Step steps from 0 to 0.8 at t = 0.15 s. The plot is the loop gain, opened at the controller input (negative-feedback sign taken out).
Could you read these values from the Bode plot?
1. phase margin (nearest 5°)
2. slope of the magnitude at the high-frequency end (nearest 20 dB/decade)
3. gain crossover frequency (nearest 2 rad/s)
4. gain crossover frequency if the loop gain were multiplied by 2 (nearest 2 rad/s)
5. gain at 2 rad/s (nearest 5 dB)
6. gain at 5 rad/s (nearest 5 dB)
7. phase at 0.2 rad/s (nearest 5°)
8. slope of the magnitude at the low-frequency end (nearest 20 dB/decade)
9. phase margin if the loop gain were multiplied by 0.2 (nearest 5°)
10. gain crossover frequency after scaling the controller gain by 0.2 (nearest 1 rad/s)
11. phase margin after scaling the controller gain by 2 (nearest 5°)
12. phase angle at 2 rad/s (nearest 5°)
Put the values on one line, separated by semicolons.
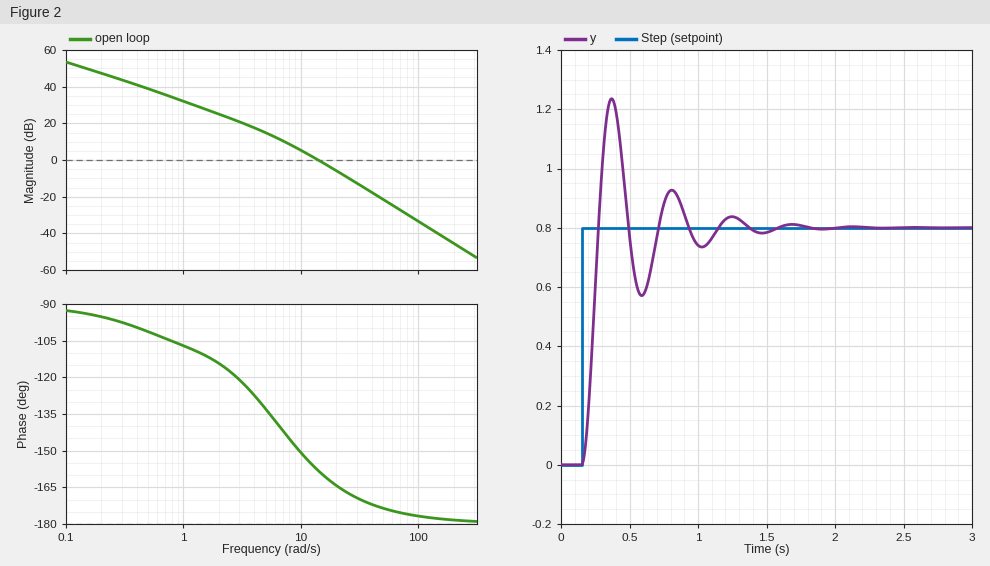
20°; -40 dB/decade; 14 rad/s; 20 rad/s; 25 dB; 15 dB; -95°; -20 dB/decade; 45°; 5 rad/s; 15°; -115°
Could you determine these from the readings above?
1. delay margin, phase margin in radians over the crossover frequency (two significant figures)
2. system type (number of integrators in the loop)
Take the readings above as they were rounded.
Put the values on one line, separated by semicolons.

0.025 s; 1
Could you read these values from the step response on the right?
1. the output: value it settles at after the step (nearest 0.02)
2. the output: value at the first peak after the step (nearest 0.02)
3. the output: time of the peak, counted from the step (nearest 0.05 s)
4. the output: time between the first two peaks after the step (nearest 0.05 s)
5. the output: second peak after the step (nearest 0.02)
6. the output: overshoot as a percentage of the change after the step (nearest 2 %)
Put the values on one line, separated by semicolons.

0.80; 1.24; 0.20 s; 0.45 s; 0.92; 54 %
